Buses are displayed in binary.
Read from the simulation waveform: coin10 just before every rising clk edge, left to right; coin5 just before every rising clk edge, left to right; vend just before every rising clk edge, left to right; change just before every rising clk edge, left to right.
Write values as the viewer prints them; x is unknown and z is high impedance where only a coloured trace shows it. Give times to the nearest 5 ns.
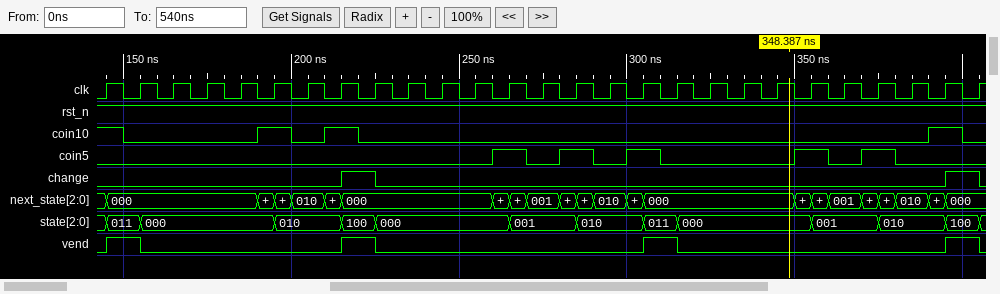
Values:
1 0 0 0 0 1 0 1 0 0 0 0 0 0 0 0 0 0 0 0 0 0 0 0 0 1 0
0 0 0 0 0 0 0 0 0 0 0 0 1 0 1 0 1 0 0 0 0 1 0 1 0 0 0
0 1 0 0 0 0 0 0 1 0 0 0 0 0 0 0 0 1 0 0 0 0 0 0 0 0 1
0 0 0 0 0 0 0 0 1 0 0 0 0 0 0 0 0 0 0 0 0 0 0 0 0 0 1
